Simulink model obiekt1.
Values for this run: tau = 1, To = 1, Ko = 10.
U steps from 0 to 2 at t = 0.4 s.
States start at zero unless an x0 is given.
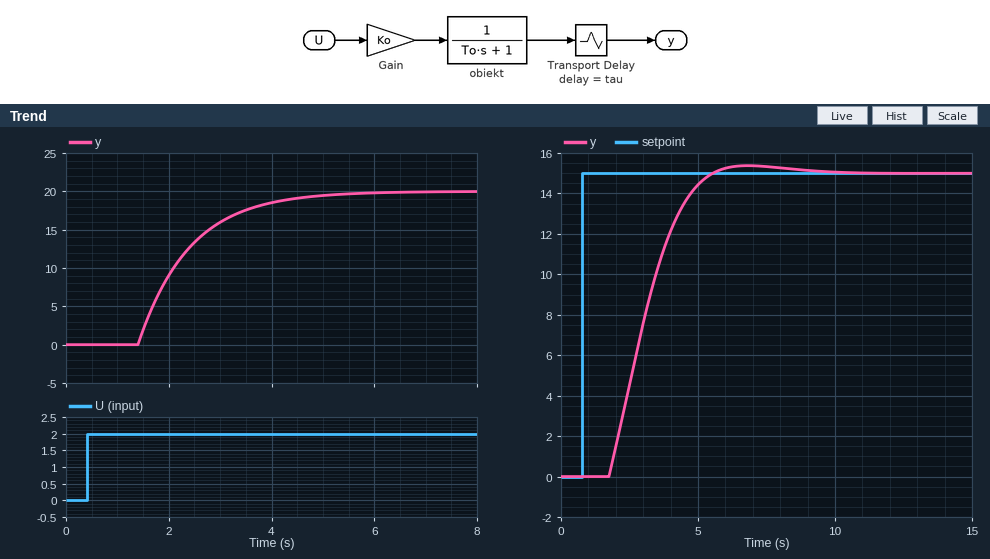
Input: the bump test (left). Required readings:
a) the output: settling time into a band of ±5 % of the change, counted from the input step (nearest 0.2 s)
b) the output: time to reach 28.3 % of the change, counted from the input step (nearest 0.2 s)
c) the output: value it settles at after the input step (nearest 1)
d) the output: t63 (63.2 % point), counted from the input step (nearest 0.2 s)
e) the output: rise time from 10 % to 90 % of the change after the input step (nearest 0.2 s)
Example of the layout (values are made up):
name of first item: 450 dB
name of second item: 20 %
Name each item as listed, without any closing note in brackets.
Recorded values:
the output: settling time into a band of ±5 % of the change, counted from the input step: 4.0 s
the output: time to reach 28.3 % of the change, counted from the input step: 1.4 s
the output: value it settles at after the input step: 20
the output: t63 (63.2 % point), counted from the input step: 2.0 s
the output: rise time from 10 % to 90 % of the change after the input step: 2.2 s
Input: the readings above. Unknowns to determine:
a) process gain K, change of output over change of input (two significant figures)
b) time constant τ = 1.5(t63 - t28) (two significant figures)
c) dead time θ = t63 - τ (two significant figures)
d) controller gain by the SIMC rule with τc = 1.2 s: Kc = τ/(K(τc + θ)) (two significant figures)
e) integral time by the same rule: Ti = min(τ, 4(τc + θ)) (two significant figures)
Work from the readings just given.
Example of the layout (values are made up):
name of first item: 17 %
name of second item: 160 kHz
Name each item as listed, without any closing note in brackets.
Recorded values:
process gain K, change of output over change of input: 10
time constant τ = 1.5(t63 - t28): 0.90 s
dead time θ = t63 - τ: 1.1 s
controller gain by the SIMC rule with τc = 1.2 s: Kc = τ/(K(τc + θ)): 0.039
integral time by the same rule: Ti = min(τ, 4(τc + θ)): 0.90 s
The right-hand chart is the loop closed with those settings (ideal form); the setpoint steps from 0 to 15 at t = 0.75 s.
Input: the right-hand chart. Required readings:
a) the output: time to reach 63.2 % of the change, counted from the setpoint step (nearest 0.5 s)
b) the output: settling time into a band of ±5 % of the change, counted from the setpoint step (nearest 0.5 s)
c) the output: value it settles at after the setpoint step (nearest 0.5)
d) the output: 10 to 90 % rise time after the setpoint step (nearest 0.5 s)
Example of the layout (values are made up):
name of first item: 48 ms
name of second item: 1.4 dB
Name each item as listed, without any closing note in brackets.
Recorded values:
the output: time to reach 63.2 % of the change, counted from the setpoint step: 2.5 s
the output: settling time into a band of ±5 % of the change, counted from the setpoint step: 4.0 s
the output: value it settles at after the setpoint step: 15.0
the output: 10 to 90 % rise time after the setpoint step: 2.5 s
